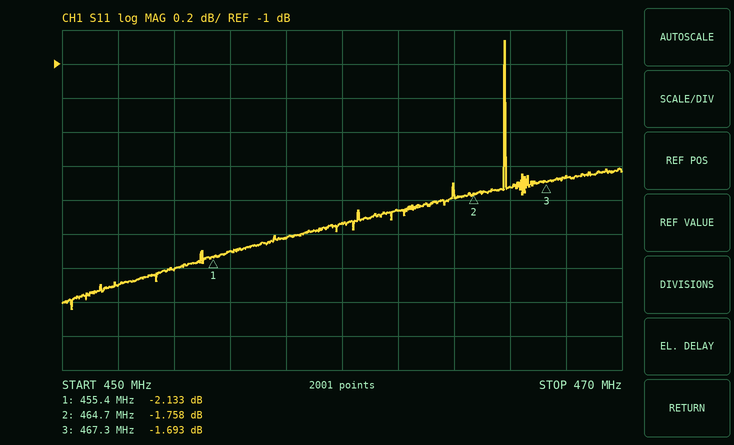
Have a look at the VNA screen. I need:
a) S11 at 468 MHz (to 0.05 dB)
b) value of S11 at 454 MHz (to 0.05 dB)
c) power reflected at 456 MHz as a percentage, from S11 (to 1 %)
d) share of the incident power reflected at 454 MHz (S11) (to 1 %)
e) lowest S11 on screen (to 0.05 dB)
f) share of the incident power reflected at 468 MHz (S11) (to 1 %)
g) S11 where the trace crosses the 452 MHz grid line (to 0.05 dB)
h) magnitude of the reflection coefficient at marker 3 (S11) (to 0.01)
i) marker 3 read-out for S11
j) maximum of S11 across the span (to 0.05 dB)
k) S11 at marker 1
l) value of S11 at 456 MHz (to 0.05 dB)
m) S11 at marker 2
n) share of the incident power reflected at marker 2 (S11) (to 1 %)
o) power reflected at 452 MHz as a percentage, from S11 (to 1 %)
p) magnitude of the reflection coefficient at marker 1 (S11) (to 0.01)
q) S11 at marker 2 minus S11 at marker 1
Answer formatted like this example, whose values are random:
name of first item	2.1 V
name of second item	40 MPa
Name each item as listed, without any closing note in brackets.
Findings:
S11 at 468 MHz	-1.65 dB
value of S11 at 454 MHz	-2.20 dB
power reflected at 456 MHz as a percentage, from S11	62 %
share of the incident power reflected at 454 MHz (S11)	60 %
lowest S11 on screen	-2.45 dB
share of the incident power reflected at 468 MHz (S11)	68 %
S11 where the trace crosses the 452 MHz grid line	-2.30 dB
magnitude of the reflection coefficient at marker 3 (S11)	0.82
marker 3 read-out for S11	-1.693 dB
maximum of S11 across the span	-0.85 dB
S11 at marker 1	-2.133 dB
value of S11 at 456 MHz	-2.10 dB
S11 at marker 2	-1.758 dB
share of the incident power reflected at marker 2 (S11)	67 %
power reflected at 452 MHz as a percentage, from S11	59 %
magnitude of the reflection coefficient at marker 1 (S11)	0.78
S11 at marker 2 minus S11 at marker 1	0.375 dB
